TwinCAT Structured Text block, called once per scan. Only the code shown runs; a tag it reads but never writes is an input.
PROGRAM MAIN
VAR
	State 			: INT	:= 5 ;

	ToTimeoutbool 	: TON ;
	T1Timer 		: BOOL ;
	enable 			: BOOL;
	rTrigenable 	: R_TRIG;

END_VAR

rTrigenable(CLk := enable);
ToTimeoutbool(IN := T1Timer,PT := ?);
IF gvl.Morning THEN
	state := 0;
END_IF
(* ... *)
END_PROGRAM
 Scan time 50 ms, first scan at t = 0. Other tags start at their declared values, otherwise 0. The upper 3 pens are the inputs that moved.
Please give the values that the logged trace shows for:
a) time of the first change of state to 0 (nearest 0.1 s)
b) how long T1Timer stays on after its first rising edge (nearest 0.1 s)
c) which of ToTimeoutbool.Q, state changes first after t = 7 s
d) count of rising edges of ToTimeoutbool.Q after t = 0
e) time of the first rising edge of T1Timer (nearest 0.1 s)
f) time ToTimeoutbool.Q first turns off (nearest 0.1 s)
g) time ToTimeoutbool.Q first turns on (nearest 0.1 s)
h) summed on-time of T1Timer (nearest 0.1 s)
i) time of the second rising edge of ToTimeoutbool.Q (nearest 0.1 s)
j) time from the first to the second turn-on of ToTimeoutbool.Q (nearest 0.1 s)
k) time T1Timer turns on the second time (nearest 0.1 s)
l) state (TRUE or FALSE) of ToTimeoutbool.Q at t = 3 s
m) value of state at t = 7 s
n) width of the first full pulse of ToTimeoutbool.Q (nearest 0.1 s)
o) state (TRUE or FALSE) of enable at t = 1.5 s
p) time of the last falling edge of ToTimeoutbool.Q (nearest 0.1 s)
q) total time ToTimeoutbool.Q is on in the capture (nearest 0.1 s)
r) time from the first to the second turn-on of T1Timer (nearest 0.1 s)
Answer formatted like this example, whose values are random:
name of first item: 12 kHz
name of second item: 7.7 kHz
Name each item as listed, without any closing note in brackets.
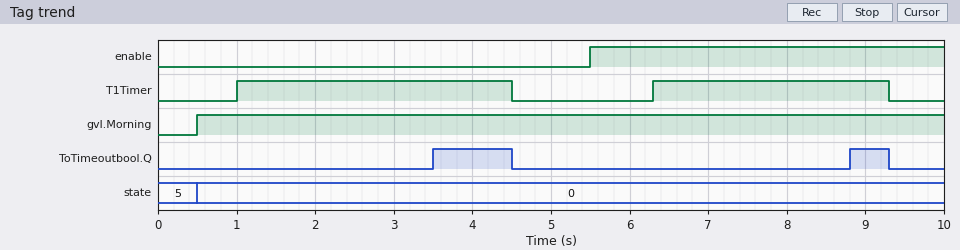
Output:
time of the first change of state to 0: 0.5 s
how long T1Timer stays on after its first rising edge: 3.5 s
which of ToTimeoutbool.Q, state changes first after t = 7 s: ToTimeoutbool.Q
count of rising edges of ToTimeoutbool.Q after t = 0: 2
time of the first rising edge of T1Timer: 1.0 s
time ToTimeoutbool.Q first turns off: 4.5 s
time ToTimeoutbool.Q first turns on: 3.5 s
summed on-time of T1Timer: 6.5 s
time of the second rising edge of ToTimeoutbool.Q: 8.8 s
time from the first to the second turn-on of ToTimeoutbool.Q: 5.3 s
time T1Timer turns on the second time: 6.3 s
state (TRUE or FALSE) of ToTimeoutbool.Q at t = 3 s: FALSE
value of state at t = 7 s: 0
width of the first full pulse of ToTimeoutbool.Q: 1.0 s
state (TRUE or FALSE) of enable at t = 1.5 s: FALSE
time of the last falling edge of ToTimeoutbool.Q: 9.3 s
total time ToTimeoutbool.Q is on in the capture: 1.5 s
time from the first to the second turn-on of T1Timer: 5.3 s
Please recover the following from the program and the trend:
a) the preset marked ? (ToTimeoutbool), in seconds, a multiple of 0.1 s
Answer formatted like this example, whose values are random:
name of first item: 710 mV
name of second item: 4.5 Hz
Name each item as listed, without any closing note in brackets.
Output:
the preset marked ? (ToTimeoutbool), in seconds, a multiple of 0.1 s: 2.5 s
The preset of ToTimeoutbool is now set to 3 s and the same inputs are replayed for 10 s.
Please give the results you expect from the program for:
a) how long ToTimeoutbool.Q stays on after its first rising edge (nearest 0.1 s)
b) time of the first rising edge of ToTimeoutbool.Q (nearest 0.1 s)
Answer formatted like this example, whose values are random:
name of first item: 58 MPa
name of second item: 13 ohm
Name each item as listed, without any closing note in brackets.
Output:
how long ToTimeoutbool.Q stays on after its first rising edge: 0.5 s
time of the first rising edge of ToTimeoutbool.Q: 4.0 s
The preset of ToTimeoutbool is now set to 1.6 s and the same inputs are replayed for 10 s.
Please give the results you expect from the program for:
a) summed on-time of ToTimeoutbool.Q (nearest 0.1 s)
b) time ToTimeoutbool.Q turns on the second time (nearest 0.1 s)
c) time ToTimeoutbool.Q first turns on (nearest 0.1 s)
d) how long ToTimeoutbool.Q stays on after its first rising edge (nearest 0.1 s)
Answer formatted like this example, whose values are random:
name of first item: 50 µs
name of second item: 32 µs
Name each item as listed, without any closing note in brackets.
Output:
summed on-time of ToTimeoutbool.Q: 3.3 s
time ToTimeoutbool.Q turns on the second time: 7.9 s
time ToTimeoutbool.Q first turns on: 2.6 s
how long ToTimeoutbool.Q stays on after its first rising edge: 1.9 s
